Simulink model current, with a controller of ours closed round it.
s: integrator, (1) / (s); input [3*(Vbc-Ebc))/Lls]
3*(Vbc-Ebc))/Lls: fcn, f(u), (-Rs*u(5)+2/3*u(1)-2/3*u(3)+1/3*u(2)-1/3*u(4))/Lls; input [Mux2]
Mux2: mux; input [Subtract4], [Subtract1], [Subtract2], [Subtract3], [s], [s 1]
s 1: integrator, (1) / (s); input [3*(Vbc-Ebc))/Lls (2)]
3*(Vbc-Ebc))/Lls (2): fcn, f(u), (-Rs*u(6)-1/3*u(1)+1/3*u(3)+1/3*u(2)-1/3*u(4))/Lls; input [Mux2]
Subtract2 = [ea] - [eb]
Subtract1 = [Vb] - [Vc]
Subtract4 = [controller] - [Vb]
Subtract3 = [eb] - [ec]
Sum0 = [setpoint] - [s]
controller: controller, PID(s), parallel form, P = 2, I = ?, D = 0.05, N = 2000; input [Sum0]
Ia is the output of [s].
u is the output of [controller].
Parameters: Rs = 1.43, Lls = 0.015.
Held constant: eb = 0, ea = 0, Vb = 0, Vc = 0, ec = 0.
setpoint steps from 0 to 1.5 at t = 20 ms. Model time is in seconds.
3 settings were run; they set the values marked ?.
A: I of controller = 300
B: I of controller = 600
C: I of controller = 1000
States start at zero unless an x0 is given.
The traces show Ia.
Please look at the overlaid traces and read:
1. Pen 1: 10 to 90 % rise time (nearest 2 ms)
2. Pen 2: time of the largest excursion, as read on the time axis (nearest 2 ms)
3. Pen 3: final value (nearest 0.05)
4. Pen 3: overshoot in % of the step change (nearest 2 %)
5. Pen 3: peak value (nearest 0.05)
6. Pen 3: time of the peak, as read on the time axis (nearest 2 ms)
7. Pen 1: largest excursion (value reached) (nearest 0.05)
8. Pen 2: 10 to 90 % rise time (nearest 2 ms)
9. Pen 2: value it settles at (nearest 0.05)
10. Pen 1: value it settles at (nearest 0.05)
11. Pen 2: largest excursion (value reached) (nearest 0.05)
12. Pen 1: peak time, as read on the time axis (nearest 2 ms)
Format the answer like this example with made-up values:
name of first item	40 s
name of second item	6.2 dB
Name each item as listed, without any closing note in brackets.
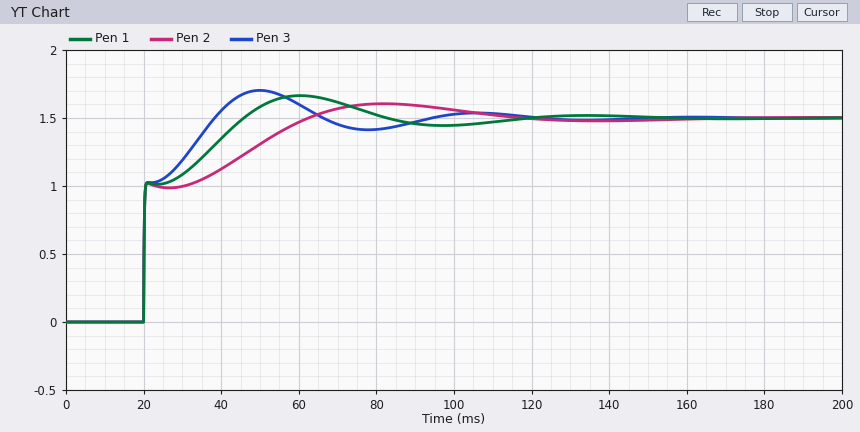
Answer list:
Pen 1: 10 to 90 % rise time	20 ms
Pen 2: time of the largest excursion, as read on the time axis	82 ms
Pen 3: final value	1.50
Pen 3: overshoot in % of the step change	14 %
Pen 3: peak value	1.70
Pen 3: time of the peak, as read on the time axis	50 ms
Pen 1: largest excursion (value reached)	1.65
Pen 2: 10 to 90 % rise time	32 ms
Pen 2: value it settles at	1.50
Pen 1: value it settles at	1.50
Pen 2: largest excursion (value reached)	1.60
Pen 1: peak time, as read on the time axis	60 ms
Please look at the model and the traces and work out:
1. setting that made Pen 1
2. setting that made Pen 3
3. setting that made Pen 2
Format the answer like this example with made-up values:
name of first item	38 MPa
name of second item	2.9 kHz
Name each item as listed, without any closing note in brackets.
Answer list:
setting that made Pen 1	B
setting that made Pen 3	C
setting that made Pen 2	A
